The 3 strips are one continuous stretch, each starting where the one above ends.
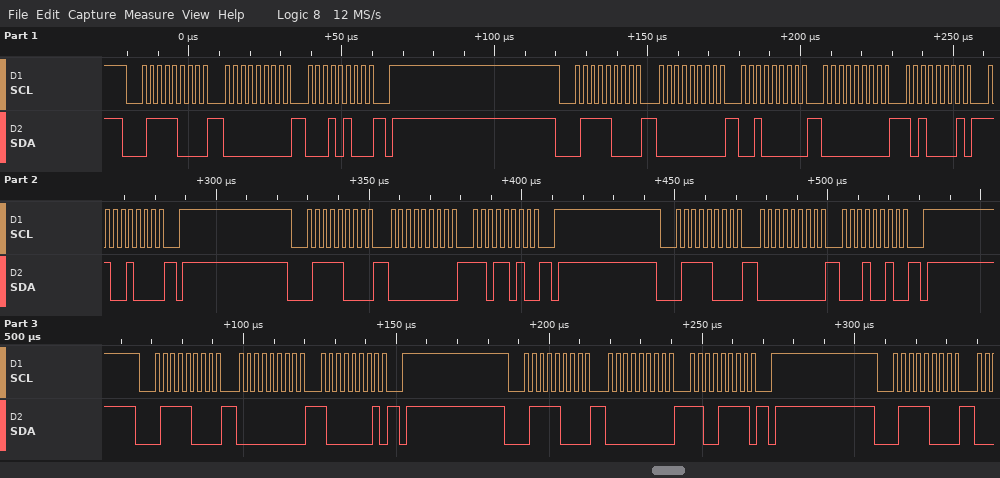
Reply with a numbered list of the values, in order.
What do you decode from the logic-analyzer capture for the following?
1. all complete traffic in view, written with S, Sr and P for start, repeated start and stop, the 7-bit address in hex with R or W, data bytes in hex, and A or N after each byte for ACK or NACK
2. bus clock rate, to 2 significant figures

1. S 3CW A 00 A 14 A P S 3CW A 00 A 20 A 00 A A1 A C8 A P S 3CW A 00 A DA A P S 3CW A 00 A 12 A P S 3CW A 00 A 81 A P S 3CW A 00 A CF A P S 3CW A
2. 400 kHz
